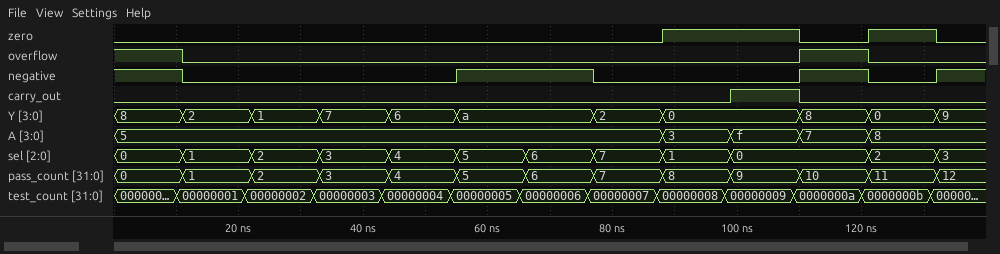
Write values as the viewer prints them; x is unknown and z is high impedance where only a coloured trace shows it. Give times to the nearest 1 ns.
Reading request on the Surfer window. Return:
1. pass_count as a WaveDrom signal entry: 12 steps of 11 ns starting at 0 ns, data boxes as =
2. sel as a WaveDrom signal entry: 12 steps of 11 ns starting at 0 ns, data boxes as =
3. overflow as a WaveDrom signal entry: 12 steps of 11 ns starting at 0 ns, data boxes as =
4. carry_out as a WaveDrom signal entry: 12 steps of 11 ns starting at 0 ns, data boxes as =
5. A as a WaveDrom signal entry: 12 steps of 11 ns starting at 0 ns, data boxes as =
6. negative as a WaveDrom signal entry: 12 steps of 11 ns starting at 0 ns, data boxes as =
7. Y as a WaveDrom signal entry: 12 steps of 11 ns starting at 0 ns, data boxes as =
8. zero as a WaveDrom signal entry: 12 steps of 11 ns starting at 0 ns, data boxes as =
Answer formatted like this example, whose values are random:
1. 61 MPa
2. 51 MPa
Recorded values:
1. {name: 'pass_count', wave: '============', data: '0 1 2 3 4 5 6 7 8 9 10 11'}
2. {name: 'sel', wave: '==========.=', data: '0 1 2 3 4 5 6 7 1 0 2'}
3. {name: 'overflow', wave: '10........10'}
4. {name: 'carry_out', wave: '0........10.'}
5. {name: 'A', wave: '=.......====', data: '5 3 f 7 8'}
6. {name: 'negative', wave: '10...1.0..10'}
7. {name: 'Y', wave: '======.==.==', data: '8 2 1 7 6 a 2 0 8 0'}
8. {name: 'zero', wave: '0.......1.01'}
